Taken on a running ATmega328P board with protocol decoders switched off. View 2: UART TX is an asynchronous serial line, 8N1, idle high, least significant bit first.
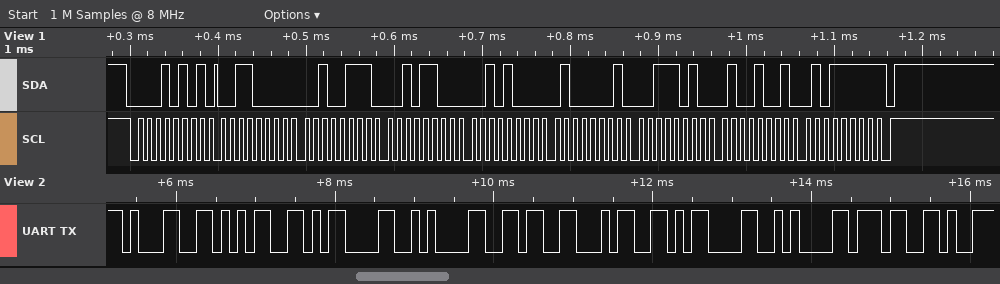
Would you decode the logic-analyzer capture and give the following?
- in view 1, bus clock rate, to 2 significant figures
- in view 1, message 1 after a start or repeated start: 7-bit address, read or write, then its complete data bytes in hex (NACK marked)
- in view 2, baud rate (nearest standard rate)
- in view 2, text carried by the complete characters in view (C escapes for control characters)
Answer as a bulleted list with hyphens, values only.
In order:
- 100 kHz
- 0x0A read: 30 27 2C 28 41 3A 49 5F NACK
- 9600 baud
- "15\r\n64\r\n7"
